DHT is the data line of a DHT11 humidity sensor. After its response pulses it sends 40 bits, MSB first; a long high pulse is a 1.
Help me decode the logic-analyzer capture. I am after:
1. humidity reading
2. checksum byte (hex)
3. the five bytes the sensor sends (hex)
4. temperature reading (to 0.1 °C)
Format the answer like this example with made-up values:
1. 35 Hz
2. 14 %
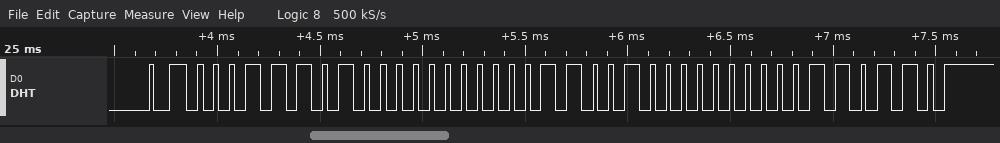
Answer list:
1. 29 %
2. 0x36
3. 1D 00 19 00 36
4. 25.0 °C
